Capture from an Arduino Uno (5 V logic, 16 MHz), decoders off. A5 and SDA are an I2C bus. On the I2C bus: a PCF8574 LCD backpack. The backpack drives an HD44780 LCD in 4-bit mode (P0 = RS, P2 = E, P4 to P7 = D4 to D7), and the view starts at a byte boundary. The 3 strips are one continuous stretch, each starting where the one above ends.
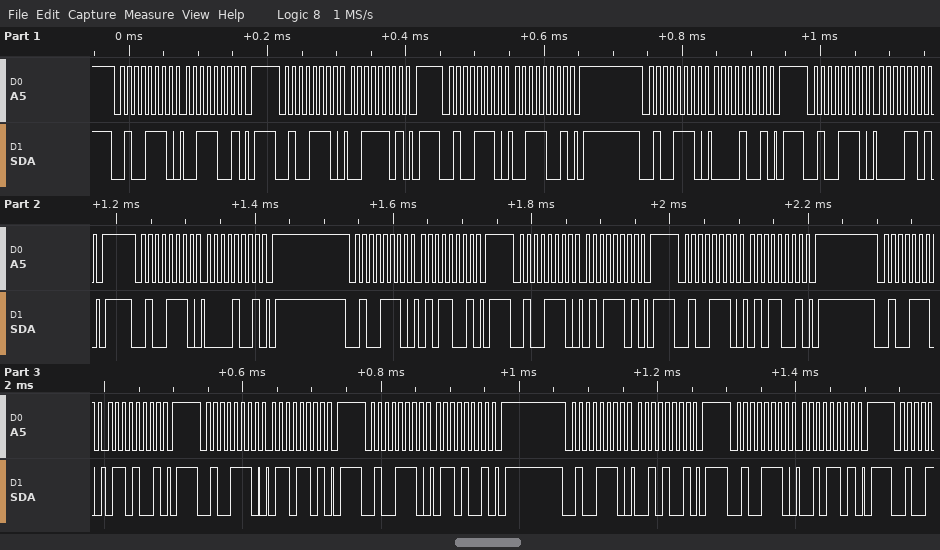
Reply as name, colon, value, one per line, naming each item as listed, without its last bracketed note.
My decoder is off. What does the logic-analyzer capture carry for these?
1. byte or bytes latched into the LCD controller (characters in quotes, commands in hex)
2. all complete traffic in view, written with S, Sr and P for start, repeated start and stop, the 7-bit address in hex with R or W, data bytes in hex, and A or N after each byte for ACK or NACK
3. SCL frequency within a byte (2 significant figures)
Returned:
byte or bytes latched into the LCD controller: '0' 'V'
all complete traffic in view, written with S, Sr and P for start, repeated start and stop, the 7-bit address in hex with R or W, data bytes in hex, and A or N after each byte for ACK or NACK: S 27W A 39 A P S 27W A 3D A P S 27W A 39 A P S 27W A 09 A P S 27W A 0D A P S 27W A 09 A P S 27W A 59 A P S 27W A 5D A P S 27W A 59 A P S 27W A 69 A P S 27W A 6D A P S 27W A 69 A P S 27W A 29 A P S 27W A 2D A P
SCL frequency within a byte: 100 kHz
